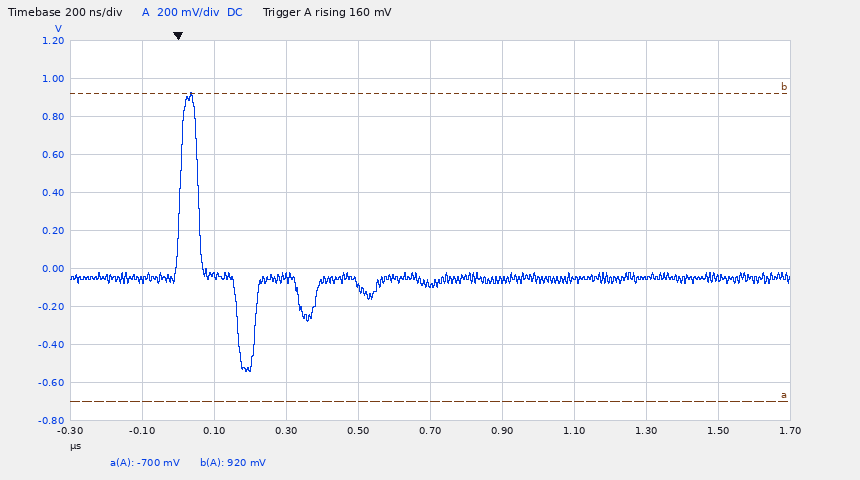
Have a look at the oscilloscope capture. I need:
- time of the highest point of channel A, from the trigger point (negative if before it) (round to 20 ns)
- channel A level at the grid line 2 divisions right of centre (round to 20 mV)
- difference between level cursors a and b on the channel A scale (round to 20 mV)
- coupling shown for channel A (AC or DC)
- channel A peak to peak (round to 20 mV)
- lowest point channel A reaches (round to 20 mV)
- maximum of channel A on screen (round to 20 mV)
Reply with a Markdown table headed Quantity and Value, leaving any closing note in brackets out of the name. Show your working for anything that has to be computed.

| Quantity | Value |
|---|---|
| time of the highest point of channel A, from the trigger point (negative if before it) | +40 ns |
| channel A level at the grid line 2 divisions right of centre | -60 mV |
| difference between level cursors a and b on the channel A scale | 1.62 V |
| coupling shown for channel A | DC |
| channel A peak to peak | 920 mV − (-540 mV) = 1.46 V |
| lowest point channel A reaches | -540 mV |
| maximum of channel A on screen | 920 mV |
